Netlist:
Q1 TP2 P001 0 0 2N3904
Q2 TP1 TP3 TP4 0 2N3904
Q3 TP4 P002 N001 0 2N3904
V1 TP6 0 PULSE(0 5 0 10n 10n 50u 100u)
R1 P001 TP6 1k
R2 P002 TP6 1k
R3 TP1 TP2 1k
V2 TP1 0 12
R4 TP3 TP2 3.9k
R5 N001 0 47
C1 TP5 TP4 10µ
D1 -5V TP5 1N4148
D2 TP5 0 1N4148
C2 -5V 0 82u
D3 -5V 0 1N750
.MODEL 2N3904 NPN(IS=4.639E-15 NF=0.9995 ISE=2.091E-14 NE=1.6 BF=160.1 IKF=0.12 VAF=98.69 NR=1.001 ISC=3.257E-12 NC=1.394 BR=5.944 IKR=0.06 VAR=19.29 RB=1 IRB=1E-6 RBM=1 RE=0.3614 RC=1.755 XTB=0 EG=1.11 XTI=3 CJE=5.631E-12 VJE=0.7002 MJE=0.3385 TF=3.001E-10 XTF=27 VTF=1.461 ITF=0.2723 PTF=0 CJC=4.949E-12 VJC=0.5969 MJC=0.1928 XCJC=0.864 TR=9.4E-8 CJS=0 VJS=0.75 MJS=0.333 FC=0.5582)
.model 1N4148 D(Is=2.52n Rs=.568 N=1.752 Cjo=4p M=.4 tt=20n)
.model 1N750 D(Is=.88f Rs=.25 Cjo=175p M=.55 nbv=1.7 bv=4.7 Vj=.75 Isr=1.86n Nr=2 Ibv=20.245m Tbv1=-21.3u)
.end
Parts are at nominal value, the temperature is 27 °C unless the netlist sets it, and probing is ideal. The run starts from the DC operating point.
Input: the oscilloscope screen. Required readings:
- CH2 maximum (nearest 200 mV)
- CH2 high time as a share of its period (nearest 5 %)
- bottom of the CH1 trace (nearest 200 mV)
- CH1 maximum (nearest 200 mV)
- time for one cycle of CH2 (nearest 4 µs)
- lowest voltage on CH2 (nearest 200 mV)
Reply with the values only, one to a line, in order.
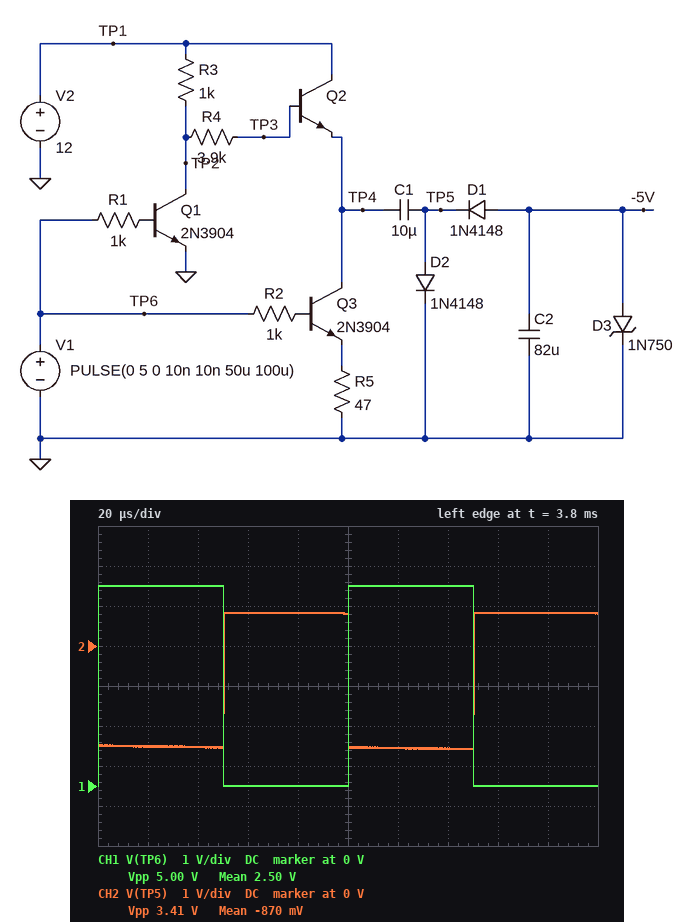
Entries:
800 mV
50 %
0 V
5.0 V
100 µs
-2.6 V
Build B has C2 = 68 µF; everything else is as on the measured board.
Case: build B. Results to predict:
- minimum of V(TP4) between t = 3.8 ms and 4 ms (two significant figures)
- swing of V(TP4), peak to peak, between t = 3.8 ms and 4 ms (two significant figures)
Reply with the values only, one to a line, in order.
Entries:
3.9 V
4.1 V
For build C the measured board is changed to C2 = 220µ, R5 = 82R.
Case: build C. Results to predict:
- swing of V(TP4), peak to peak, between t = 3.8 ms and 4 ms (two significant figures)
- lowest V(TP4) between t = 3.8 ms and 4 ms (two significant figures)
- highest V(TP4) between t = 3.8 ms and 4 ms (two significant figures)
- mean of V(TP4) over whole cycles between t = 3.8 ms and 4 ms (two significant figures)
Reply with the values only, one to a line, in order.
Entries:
2.2 V
7.2 V
9.4 V
8.3 V
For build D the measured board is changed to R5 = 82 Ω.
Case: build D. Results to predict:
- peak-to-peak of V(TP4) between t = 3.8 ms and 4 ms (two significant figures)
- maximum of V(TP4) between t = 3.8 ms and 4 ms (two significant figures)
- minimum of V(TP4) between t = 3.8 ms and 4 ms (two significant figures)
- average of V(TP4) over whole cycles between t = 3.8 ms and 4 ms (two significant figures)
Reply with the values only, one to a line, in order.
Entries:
2.9 V
9.4 V
6.5 V
7.9 V
